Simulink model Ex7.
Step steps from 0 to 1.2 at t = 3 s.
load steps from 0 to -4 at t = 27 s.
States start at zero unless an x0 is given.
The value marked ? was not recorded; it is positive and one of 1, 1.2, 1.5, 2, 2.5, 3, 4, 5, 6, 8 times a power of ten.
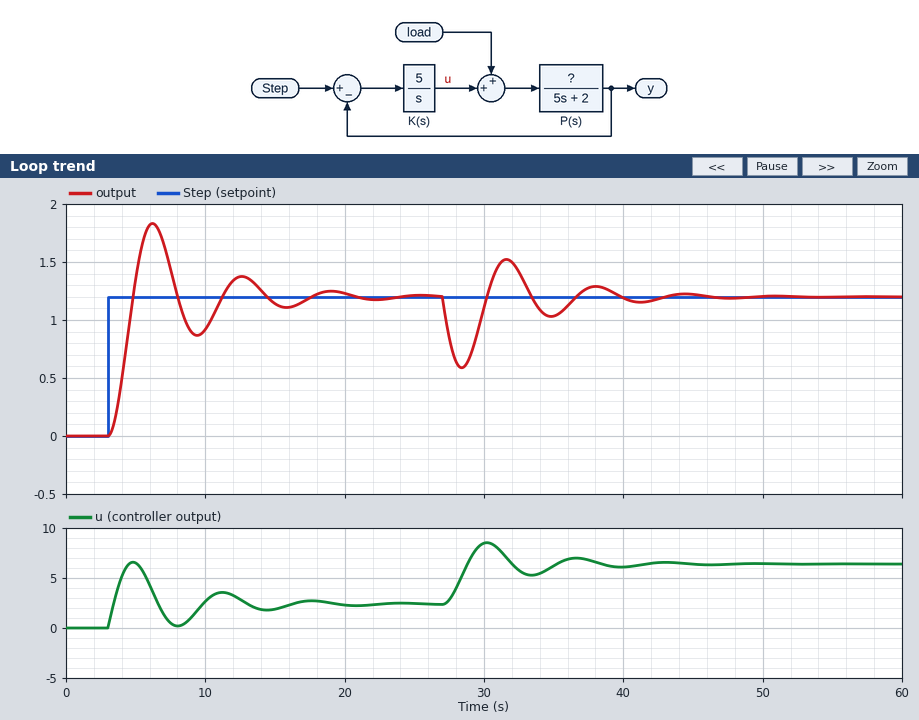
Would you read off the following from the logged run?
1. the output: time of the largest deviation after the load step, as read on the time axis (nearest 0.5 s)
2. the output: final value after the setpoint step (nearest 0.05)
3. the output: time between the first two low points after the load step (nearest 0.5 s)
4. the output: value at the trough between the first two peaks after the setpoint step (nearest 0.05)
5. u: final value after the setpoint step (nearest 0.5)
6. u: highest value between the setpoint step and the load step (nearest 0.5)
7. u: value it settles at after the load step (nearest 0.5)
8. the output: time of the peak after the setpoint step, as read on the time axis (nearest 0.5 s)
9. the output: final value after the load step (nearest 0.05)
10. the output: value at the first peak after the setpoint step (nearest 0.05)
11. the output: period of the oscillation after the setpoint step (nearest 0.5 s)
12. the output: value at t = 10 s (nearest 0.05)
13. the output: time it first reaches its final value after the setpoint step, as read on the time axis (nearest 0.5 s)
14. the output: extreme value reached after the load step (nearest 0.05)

28.5 s
1.20
6.5 s
0.85
2.5
6.5
6.5
6.0 s
1.20
1.85
6.5 s
0.90
5.0 s
0.60
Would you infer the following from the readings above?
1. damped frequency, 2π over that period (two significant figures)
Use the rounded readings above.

0.97 rad/s
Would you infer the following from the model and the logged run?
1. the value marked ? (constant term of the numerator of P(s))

1
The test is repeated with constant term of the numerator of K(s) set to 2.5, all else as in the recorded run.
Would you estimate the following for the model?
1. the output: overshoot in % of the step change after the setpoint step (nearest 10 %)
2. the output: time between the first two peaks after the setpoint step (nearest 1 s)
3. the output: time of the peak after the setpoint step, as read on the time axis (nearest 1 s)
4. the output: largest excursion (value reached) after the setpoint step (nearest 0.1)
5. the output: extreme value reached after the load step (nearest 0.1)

40 %
9 s
8 s
1.7
0.4
